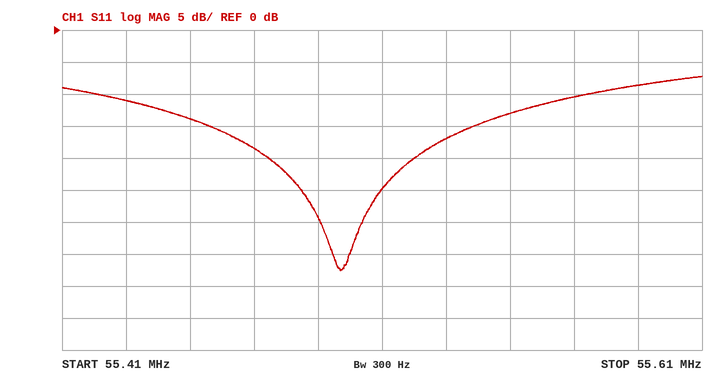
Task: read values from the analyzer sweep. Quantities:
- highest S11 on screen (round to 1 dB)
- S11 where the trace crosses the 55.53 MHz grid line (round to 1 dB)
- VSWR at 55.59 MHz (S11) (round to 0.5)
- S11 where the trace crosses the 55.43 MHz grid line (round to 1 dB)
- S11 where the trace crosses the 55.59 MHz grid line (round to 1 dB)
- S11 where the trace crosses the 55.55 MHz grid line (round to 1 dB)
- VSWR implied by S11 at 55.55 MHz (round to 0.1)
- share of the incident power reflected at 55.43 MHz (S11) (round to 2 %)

-7 dB
-17 dB
2.0
-11 dB
-9 dB
-13 dB
1.6
8 %
